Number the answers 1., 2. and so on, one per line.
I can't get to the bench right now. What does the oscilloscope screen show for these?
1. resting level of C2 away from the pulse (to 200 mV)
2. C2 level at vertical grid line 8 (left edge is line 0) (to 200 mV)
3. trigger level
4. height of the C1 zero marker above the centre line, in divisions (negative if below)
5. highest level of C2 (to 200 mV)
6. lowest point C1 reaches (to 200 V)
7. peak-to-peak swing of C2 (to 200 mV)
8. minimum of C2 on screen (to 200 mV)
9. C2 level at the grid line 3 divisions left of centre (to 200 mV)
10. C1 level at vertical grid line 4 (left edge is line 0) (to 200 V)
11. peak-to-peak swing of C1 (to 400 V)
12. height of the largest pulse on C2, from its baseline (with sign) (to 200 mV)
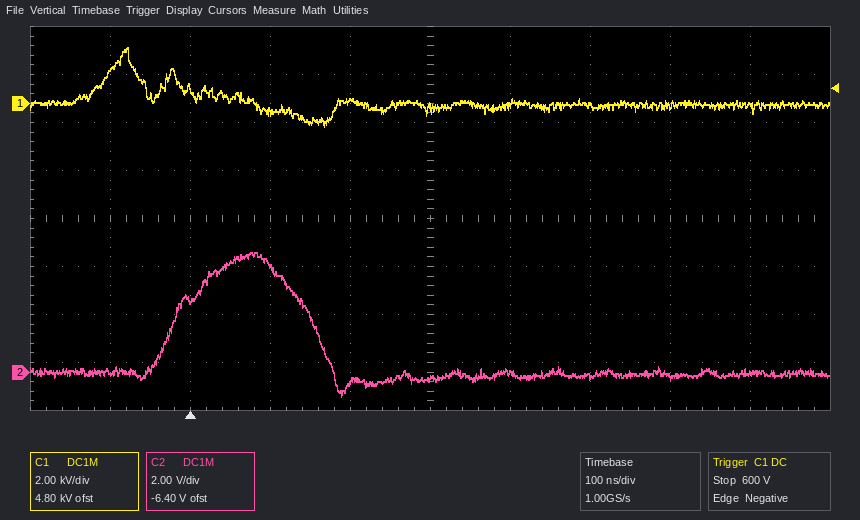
1. 0.0 V
2. -200 mV
3. 600 V
4. +2.4 div
5. 5.0 V
6. -1.0 kV
7. 6.0 V
8. -1.0 V
9. 3.0 V
10. 0.0 kV
11. 3.2 kV
12. +5.0 V
